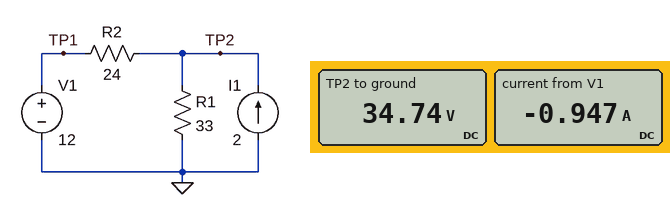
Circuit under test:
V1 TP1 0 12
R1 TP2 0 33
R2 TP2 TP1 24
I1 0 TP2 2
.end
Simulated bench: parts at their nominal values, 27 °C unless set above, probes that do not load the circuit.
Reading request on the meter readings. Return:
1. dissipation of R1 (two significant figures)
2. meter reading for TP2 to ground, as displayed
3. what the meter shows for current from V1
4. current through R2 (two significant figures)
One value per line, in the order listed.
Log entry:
37 W
34.74 V
-0.947 A
950 mA
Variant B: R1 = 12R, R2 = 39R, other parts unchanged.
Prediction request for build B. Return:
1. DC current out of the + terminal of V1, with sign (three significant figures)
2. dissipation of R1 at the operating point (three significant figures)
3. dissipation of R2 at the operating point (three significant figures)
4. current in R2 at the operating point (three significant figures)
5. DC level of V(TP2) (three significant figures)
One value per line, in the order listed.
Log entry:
-235 mA
37.4 W
2.16 W
235 mA
21.2 V
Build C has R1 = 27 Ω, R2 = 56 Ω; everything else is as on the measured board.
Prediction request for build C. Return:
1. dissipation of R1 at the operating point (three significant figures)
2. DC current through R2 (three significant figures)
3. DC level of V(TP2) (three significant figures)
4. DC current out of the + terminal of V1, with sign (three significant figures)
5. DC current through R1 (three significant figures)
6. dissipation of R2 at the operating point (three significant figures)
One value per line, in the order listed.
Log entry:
60.3 W
506 mA
40.3 V
-506 mA
1.49 A
14.3 W
